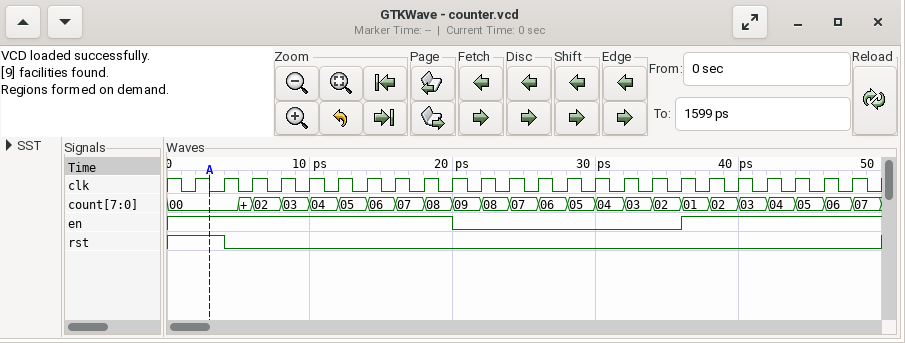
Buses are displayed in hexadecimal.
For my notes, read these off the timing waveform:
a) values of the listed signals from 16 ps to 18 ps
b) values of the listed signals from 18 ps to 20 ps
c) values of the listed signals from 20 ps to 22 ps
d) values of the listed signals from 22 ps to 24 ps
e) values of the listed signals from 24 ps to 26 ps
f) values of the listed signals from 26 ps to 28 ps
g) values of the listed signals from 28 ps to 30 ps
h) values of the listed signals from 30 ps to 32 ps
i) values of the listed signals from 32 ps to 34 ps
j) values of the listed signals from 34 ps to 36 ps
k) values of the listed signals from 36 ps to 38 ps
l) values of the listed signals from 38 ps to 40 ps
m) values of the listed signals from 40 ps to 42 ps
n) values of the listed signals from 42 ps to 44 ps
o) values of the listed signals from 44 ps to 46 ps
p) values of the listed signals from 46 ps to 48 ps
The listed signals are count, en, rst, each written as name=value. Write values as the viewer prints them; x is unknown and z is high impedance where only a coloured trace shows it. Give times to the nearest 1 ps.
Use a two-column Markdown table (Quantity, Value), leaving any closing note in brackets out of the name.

| Quantity | Value |
|---|---|
| values of the listed signals from 16 ps to 18 ps | count=07, en=1, rst=0 |
| values of the listed signals from 18 ps to 20 ps | count=08, en=1, rst=0 |
| values of the listed signals from 20 ps to 22 ps | count=09, en=0, rst=0 |
| values of the listed signals from 22 ps to 24 ps | count=08, en=0, rst=0 |
| values of the listed signals from 24 ps to 26 ps | count=07, en=0, rst=0 |
| values of the listed signals from 26 ps to 28 ps | count=06, en=0, rst=0 |
| values of the listed signals from 28 ps to 30 ps | count=05, en=0, rst=0 |
| values of the listed signals from 30 ps to 32 ps | count=04, en=0, rst=0 |
| values of the listed signals from 32 ps to 34 ps | count=03, en=0, rst=0 |
| values of the listed signals from 34 ps to 36 ps | count=02, en=0, rst=0 |
| values of the listed signals from 36 ps to 38 ps | count=01, en=1, rst=0 |
| values of the listed signals from 38 ps to 40 ps | count=02, en=1, rst=0 |
| values of the listed signals from 40 ps to 42 ps | count=03, en=1, rst=0 |
| values of the listed signals from 42 ps to 44 ps | count=04, en=1, rst=0 |
| values of the listed signals from 44 ps to 46 ps | count=05, en=1, rst=0 |
| values of the listed signals from 46 ps to 48 ps | count=06, en=1, rst=0 |
